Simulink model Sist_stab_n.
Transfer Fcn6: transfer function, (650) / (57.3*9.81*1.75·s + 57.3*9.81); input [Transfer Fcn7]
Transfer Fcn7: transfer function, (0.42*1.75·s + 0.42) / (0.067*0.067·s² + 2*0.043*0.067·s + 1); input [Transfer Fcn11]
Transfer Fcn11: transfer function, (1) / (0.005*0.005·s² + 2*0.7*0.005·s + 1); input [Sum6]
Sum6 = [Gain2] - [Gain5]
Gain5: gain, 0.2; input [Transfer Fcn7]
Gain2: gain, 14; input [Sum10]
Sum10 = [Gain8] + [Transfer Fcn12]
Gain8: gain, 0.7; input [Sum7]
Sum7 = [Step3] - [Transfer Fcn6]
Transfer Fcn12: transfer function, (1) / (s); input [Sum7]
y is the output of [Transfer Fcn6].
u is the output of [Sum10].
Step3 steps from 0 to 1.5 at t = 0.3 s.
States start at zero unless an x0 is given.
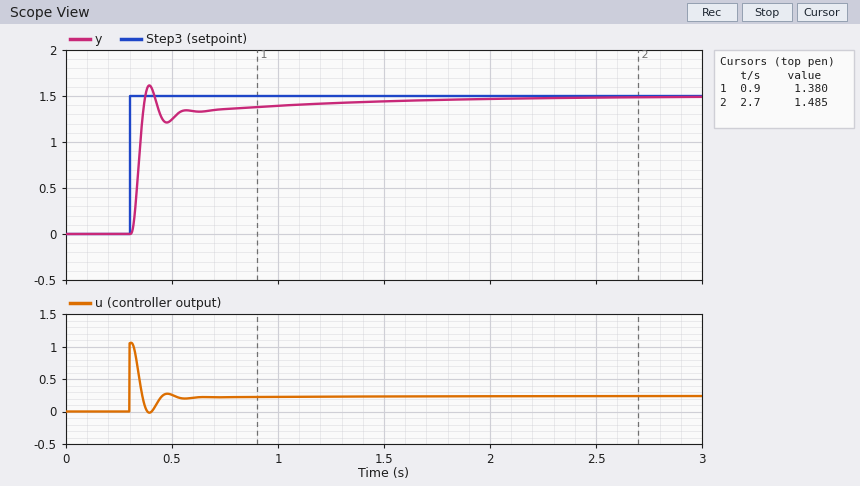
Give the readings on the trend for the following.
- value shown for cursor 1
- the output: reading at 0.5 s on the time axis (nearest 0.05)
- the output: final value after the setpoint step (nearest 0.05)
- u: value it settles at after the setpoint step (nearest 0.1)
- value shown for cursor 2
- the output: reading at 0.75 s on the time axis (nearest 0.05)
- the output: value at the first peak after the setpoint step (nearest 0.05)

1.380
1.25
1.50
0.2
1.485
1.35
1.60
